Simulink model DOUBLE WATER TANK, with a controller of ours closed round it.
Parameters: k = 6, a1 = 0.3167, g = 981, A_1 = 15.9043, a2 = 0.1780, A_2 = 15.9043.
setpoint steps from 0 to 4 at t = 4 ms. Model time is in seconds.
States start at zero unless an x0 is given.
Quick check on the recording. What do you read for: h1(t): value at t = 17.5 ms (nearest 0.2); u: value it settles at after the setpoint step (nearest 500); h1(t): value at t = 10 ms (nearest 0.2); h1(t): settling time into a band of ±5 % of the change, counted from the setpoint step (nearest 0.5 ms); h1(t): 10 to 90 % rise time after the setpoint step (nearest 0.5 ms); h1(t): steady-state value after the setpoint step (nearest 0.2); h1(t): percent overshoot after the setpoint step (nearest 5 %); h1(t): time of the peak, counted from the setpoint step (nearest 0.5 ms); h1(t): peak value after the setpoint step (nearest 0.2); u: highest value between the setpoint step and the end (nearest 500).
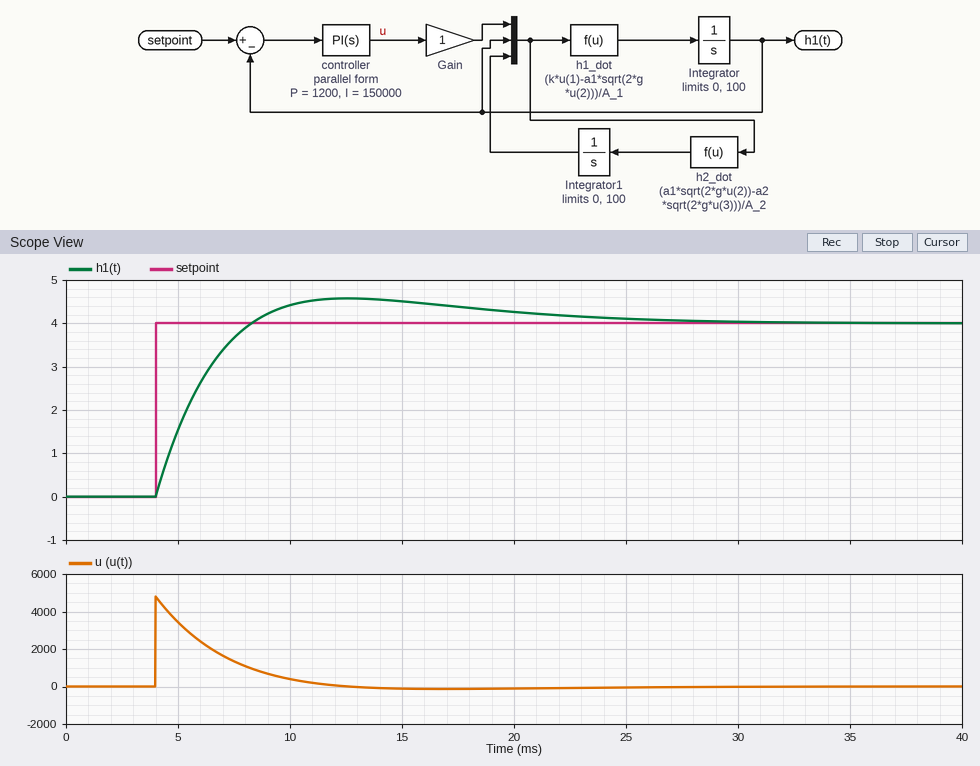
4.4
0
4.4
17.5 ms
3.0 ms
4.0
15 %
8.5 ms
4.6
5000
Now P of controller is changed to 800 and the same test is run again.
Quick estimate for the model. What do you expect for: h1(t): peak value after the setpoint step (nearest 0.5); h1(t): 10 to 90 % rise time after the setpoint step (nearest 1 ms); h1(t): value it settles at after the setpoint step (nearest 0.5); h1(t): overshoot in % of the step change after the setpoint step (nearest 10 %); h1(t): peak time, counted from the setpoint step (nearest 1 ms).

5.0
4 ms
4.0
20 %
10 ms
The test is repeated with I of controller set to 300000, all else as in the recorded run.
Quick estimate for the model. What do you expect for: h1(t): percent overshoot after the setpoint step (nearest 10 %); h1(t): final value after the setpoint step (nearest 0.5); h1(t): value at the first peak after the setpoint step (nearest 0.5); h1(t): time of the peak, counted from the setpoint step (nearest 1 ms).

20 %
4.0
5.0
7 ms
